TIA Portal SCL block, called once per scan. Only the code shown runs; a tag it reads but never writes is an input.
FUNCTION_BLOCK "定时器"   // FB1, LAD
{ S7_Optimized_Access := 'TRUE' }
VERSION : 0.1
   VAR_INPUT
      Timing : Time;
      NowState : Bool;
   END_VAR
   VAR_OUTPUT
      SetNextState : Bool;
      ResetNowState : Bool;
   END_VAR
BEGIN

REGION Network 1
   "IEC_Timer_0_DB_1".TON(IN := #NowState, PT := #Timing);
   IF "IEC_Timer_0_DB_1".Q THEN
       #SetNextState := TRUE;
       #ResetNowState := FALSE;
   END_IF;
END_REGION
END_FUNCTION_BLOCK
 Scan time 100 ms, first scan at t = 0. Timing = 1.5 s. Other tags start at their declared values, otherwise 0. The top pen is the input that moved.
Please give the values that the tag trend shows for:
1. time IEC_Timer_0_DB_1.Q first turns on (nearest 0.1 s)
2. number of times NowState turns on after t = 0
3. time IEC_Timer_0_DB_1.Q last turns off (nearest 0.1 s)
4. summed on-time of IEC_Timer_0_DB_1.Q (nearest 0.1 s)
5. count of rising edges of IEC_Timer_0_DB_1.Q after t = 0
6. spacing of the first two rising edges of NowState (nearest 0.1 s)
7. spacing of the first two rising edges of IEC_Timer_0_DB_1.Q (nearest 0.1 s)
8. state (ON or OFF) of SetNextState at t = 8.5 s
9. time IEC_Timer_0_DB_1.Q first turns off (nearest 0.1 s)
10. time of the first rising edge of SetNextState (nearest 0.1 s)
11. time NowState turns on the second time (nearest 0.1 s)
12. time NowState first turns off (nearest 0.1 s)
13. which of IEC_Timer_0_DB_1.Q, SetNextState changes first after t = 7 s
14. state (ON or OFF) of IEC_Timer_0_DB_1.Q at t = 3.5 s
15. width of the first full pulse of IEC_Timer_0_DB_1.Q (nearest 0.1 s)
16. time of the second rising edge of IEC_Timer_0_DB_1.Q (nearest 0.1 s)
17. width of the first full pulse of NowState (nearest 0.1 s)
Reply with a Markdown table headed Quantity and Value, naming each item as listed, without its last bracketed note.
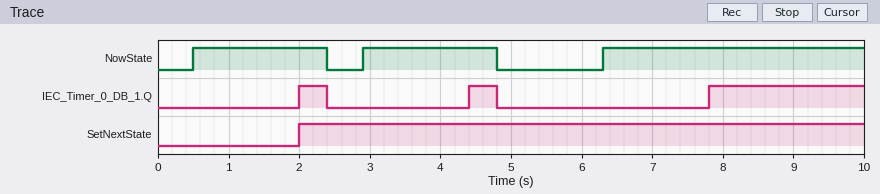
| Quantity | Value |
|---|---|
| time IEC_Timer_0_DB_1.Q first turns on | 2.0 s |
| number of times NowState turns on after t = 0 | 3 |
| time IEC_Timer_0_DB_1.Q last turns off | 4.8 s |
| summed on-time of IEC_Timer_0_DB_1.Q | 3.0 s |
| count of rising edges of IEC_Timer_0_DB_1.Q after t = 0 | 3 |
| spacing of the first two rising edges of NowState | 2.4 s |
| spacing of the first two rising edges of IEC_Timer_0_DB_1.Q | 2.4 s |
| state (ON or OFF) of SetNextState at t = 8.5 s | ON |
| time IEC_Timer_0_DB_1.Q first turns off | 2.4 s |
| time of the first rising edge of SetNextState | 2.0 s |
| time NowState turns on the second time | 2.9 s |
| time NowState first turns off | 2.4 s |
| which of IEC_Timer_0_DB_1.Q, SetNextState changes first after t = 7 s | IEC_Timer_0_DB_1.Q |
| state (ON or OFF) of IEC_Timer_0_DB_1.Q at t = 3.5 s | OFF |
| width of the first full pulse of IEC_Timer_0_DB_1.Q | 0.4 s |
| time of the second rising edge of IEC_Timer_0_DB_1.Q | 4.4 s |
| width of the first full pulse of NowState | 1.9 s |
